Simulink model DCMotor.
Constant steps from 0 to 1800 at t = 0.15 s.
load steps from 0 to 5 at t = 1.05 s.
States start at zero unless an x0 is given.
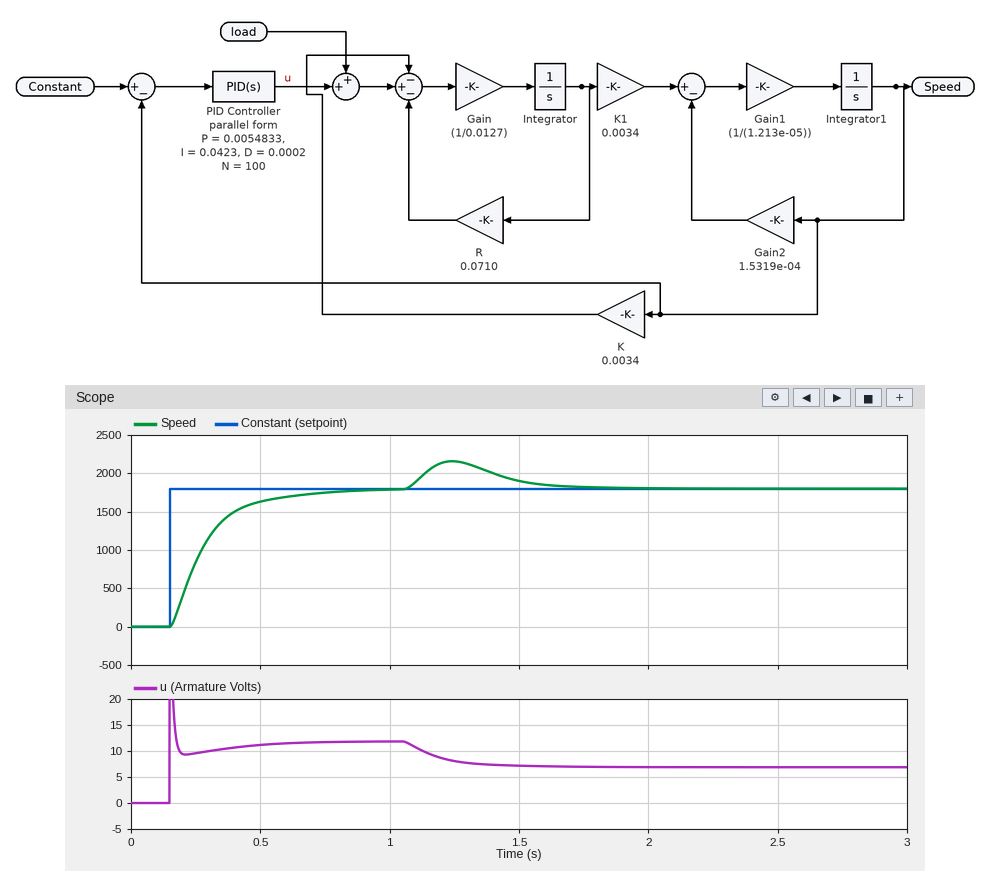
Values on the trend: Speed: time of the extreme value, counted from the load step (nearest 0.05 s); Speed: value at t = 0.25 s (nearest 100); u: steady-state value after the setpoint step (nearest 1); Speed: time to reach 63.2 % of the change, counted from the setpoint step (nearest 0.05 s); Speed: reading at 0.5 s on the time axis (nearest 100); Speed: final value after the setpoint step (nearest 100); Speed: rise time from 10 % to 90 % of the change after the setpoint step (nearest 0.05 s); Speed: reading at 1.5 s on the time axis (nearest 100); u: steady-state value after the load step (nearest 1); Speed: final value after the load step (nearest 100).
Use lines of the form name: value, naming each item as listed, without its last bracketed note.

Speed: time of the extreme value, counted from the load step: 0.20 s
Speed: value at t = 0.25 s: 800
u: steady-state value after the setpoint step: 12
Speed: time to reach 63.2 % of the change, counted from the setpoint step: 0.15 s
Speed: reading at 0.5 s on the time axis: 1600
Speed: final value after the setpoint step: 1800
Speed: rise time from 10 % to 90 % of the change after the setpoint step: 0.30 s
Speed: reading at 1.5 s on the time axis: 1900
u: steady-state value after the load step: 7
Speed: final value after the load step: 1800
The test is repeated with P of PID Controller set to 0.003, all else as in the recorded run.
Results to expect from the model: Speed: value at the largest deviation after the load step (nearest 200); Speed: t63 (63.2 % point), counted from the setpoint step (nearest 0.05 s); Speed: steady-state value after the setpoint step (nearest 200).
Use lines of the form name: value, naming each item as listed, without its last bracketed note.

Speed: value at the largest deviation after the load step: 2200
Speed: t63 (63.2 % point), counted from the setpoint step: 0.20 s
Speed: steady-state value after the setpoint step: 1800
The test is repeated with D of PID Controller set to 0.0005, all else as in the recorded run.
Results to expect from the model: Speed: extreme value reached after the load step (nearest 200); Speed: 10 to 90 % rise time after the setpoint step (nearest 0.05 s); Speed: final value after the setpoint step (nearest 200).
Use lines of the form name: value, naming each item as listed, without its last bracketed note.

Speed: extreme value reached after the load step: 2200
Speed: 10 to 90 % rise time after the setpoint step: 0.40 s
Speed: final value after the setpoint step: 1800
